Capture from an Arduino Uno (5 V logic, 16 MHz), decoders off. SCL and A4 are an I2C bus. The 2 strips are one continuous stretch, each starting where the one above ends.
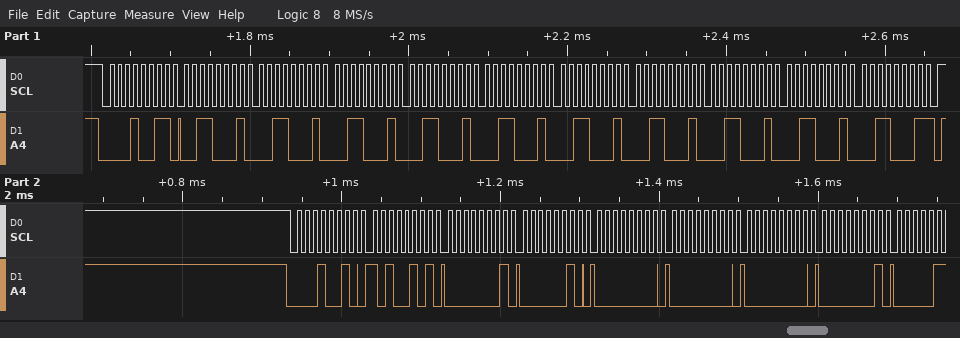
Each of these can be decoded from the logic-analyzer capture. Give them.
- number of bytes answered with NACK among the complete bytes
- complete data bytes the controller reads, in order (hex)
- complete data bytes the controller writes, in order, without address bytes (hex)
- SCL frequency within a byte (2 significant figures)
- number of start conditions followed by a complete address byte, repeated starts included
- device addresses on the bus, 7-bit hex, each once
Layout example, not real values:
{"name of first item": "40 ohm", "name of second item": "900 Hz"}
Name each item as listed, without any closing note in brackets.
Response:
{"number of bytes answered with NACK among the complete bytes": "1", "complete data bytes the controller reads, in order": "31 31 31 31 31 31 31 31 31 31", "complete data bytes the controller writes, in order, without address bytes": "A5 01 02 00 00 00 01", "SCL frequency within a byte": "100 kHz", "number of start conditions followed by a complete address byte, repeated starts included": "2", "device addresses on the bus, 7-bit hex, each once": "0x09"}
